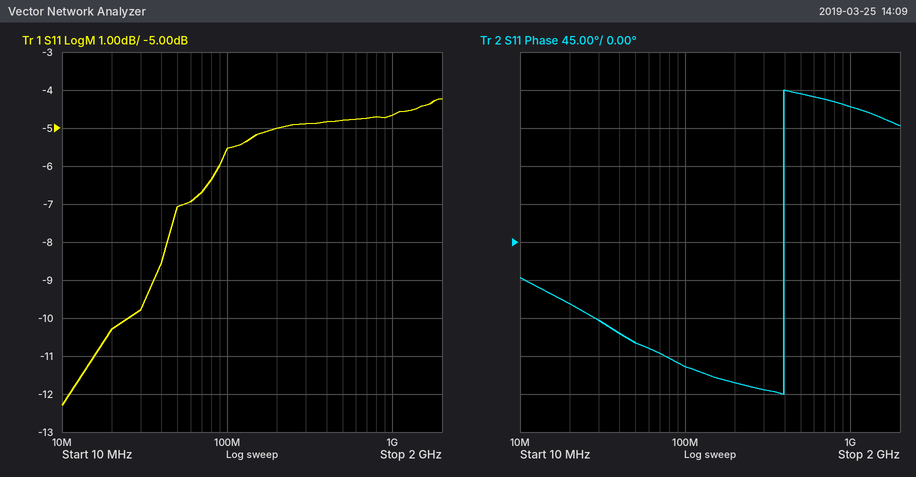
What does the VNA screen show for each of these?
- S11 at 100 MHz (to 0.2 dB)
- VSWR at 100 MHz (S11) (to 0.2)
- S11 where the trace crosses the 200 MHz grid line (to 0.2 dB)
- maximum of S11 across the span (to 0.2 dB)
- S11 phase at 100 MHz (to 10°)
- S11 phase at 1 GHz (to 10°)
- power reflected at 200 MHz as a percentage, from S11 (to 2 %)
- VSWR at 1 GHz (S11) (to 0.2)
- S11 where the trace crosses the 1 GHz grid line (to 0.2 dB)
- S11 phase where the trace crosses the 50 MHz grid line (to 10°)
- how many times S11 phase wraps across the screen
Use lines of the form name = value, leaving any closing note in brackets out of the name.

S11 at 100 MHz = -5.6 dB
VSWR at 100 MHz (S11) = 3.2
S11 where the trace crosses the 200 MHz grid line = -5.0 dB
maximum of S11 across the span = -4.2 dB
S11 phase at 100 MHz = -150°
S11 phase at 1 GHz = 160°
power reflected at 200 MHz as a percentage, from S11 = 32 %
VSWR at 1 GHz (S11) = 3.8
S11 where the trace crosses the 1 GHz grid line = -4.6 dB
S11 phase where the trace crosses the 50 MHz grid line = -120°
how many times S11 phase wraps across the screen = 1
